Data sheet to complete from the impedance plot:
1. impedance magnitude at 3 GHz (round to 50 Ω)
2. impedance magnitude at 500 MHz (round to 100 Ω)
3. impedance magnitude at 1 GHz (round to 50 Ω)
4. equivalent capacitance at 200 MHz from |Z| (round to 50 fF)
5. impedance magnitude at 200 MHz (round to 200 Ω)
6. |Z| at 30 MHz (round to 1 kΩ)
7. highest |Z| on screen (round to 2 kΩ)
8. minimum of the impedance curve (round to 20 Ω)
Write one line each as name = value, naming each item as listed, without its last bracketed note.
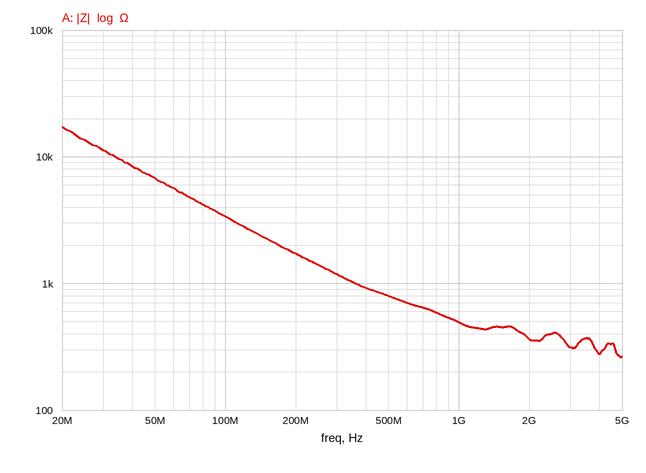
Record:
impedance magnitude at 3 GHz = 300 Ω
impedance magnitude at 500 MHz = 800 Ω
impedance magnitude at 1 GHz = 500 Ω
equivalent capacitance at 200 MHz from |Z| = 450 fF
impedance magnitude at 200 MHz = 1.8 kΩ
|Z| at 30 MHz = 11 kΩ
highest |Z| on screen = 18 kΩ
minimum of the impedance curve = 260 Ω
